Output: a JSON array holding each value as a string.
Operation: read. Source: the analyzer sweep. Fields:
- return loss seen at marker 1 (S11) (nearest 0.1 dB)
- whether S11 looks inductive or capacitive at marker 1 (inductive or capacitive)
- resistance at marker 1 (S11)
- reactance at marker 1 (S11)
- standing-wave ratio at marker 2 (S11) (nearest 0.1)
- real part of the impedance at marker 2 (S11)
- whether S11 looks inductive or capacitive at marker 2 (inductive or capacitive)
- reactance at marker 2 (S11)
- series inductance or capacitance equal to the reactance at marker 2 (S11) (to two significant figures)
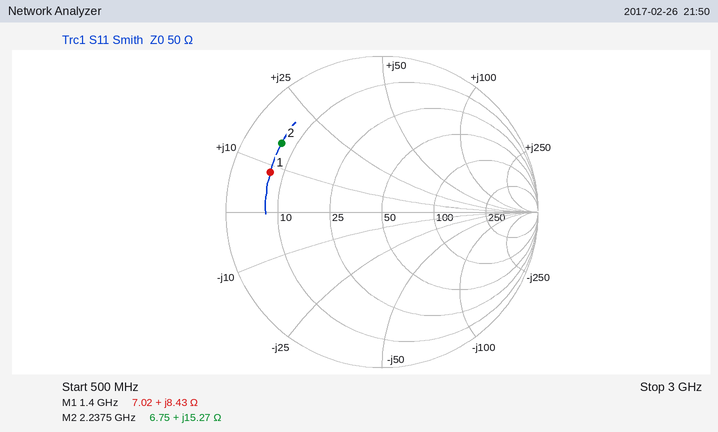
["2.4 dB", "inductive", "7.02 Ω", "+8.43 Ω", "8.1", "6.75 Ω", "inductive", "+15.27 Ω", "1.1 nH"]
